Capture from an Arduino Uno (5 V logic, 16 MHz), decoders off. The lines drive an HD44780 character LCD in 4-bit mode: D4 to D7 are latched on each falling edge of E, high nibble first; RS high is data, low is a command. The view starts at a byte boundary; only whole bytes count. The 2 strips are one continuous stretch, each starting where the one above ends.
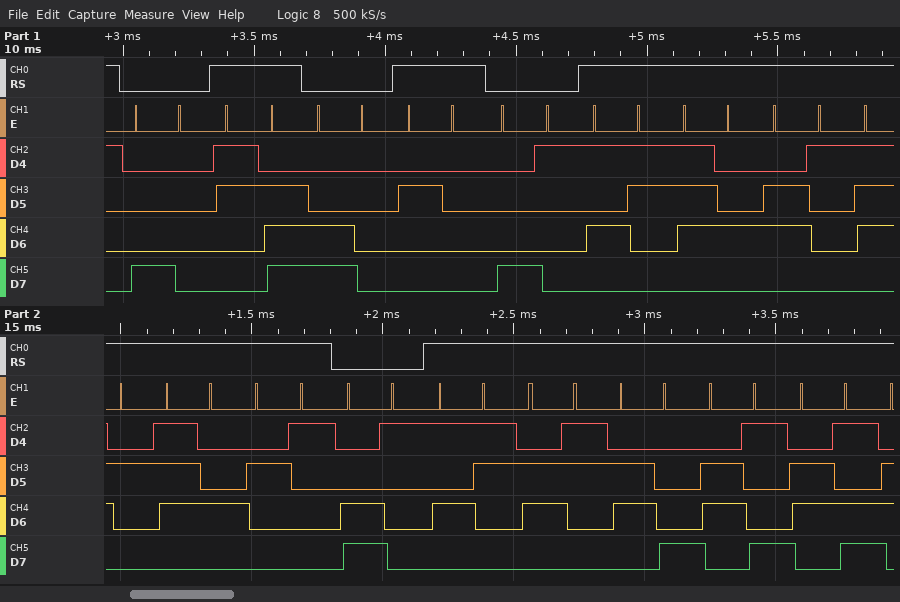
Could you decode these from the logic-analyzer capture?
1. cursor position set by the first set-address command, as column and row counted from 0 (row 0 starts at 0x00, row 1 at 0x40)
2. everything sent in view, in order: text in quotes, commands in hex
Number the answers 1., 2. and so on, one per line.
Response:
1. column 0, row 0
2. 0x80 ">" 0xC0 " " 0x81 "Start!" 0xC1 "Schim"
